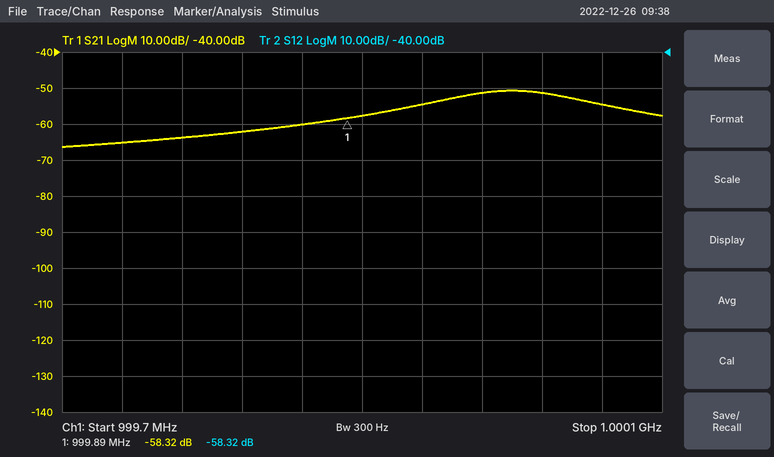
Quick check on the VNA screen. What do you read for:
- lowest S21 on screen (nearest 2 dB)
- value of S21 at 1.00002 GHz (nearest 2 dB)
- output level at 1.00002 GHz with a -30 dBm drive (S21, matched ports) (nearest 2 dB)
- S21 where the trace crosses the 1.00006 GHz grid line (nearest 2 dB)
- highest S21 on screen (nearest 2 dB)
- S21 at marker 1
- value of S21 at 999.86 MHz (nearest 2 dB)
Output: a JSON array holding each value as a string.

["-66 dB", "-52 dB", "-82 dBm", "-54 dB", "-50 dB", "-58.32 dB", "-60 dB"]
